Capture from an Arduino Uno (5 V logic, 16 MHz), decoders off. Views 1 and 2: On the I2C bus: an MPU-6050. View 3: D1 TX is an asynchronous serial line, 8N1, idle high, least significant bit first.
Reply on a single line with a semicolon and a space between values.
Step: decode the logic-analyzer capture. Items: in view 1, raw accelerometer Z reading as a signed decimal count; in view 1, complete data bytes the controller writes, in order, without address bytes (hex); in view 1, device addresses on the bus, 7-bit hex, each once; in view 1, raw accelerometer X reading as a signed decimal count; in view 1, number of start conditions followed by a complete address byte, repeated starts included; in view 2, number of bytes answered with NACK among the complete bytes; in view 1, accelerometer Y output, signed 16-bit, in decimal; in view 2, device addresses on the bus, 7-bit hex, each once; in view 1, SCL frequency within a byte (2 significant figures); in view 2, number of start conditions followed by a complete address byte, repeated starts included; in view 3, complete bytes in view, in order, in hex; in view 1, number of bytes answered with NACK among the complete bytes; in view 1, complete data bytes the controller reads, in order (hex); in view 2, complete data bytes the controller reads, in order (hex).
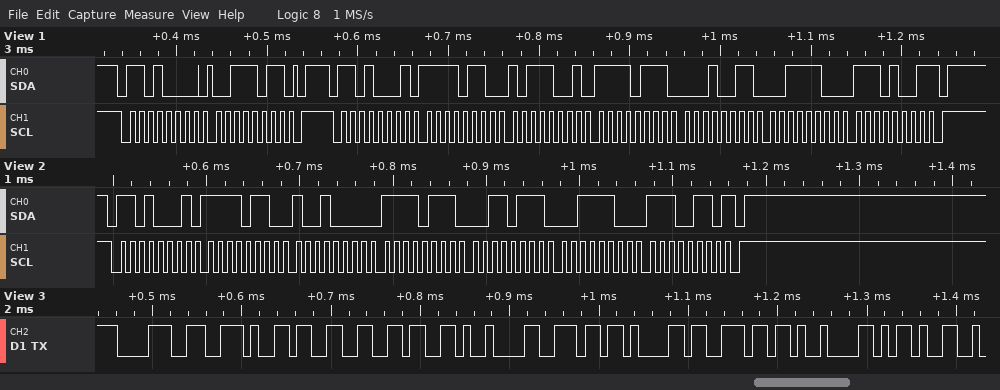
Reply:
15593; 3B; 0x68; -2375; 2; 1; -2285; 0x68; 100 kHz; 1; 38 2E 33 36 09 6E 61 6E 09 2D; 1; F6 B9 F7 13 3C E9; F6 90 F7 37 3C E6
